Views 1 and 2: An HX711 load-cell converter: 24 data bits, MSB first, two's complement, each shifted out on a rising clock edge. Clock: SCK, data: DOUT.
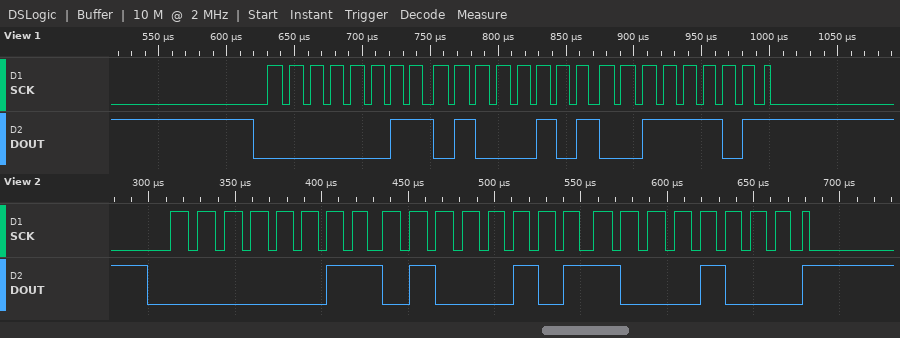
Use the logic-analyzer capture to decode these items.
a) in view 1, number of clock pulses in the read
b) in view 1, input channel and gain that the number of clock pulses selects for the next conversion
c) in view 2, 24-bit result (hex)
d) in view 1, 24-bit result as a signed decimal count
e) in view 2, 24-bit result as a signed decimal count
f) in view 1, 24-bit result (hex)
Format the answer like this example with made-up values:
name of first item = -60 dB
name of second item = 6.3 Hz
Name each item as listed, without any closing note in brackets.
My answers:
in view 1, number of clock pulses in the read = 25
in view 1, input channel and gain that the number of clock pulses selects for the next conversion = channel A, gain 128
in view 2, 24-bit result = 0x034588
in view 1, 24-bit result as a signed decimal count = 214333
in view 2, 24-bit result as a signed decimal count = 214408
in view 1, 24-bit result = 0x03453D
